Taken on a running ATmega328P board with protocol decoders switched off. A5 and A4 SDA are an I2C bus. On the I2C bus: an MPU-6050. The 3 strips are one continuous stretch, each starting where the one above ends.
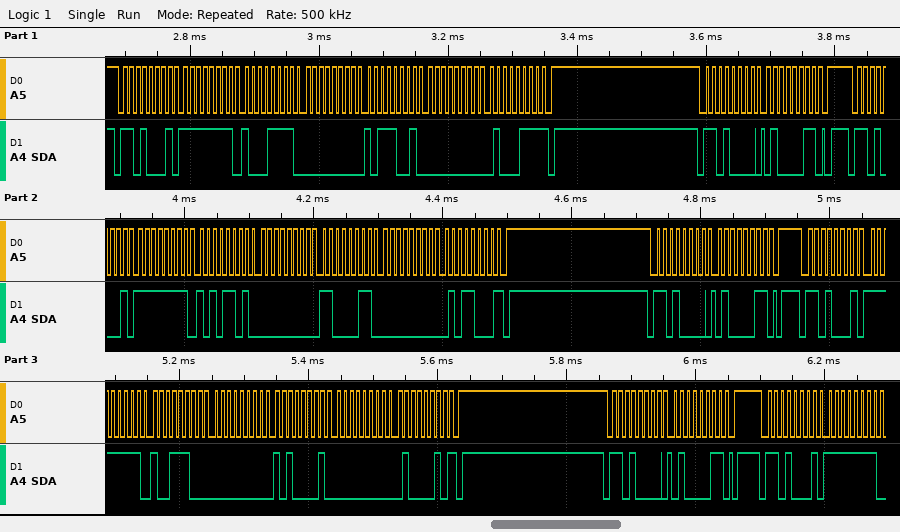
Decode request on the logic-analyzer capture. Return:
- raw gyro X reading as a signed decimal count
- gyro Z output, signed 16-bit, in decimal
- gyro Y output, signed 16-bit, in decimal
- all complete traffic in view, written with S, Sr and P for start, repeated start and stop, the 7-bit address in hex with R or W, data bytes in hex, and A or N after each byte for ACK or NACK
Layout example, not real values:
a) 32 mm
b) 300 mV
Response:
a) -83
b) 88
c) 195
d) S 68R A FF A 8F A 00 A B9 A 00 A 47 N P S 68W A 43 A P S 68R A FF A AD A 00 A C3 A 00 A 58 N P S 68W A 43 A P S 68R A FF A 9C A 00 A A1 A 00 A 42 N P S 68W A 43 A P S 68R A FF A
